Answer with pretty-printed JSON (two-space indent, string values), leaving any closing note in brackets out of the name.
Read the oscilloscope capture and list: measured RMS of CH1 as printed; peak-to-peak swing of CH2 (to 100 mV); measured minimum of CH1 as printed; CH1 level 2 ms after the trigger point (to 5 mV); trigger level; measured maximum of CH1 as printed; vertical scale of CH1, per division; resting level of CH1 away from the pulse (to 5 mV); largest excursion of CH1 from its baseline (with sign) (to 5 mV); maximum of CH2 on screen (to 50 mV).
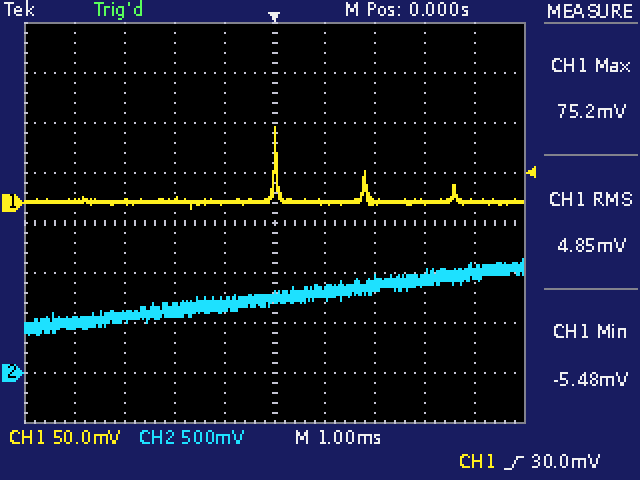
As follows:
{
  "measured RMS of CH1 as printed": "4.85 mV",
  "peak-to-peak swing of CH2": "800 mV",
  "measured minimum of CH1 as printed": "-5.48 mV",
  "CH1 level 2 ms after the trigger point": "0 mV",
  "trigger level": "30.0 mV",
  "measured maximum of CH1 as printed": "75.2 mV",
  "vertical scale of CH1, per division": "50 mV",
  "resting level of CH1 away from the pulse": "0 mV",
  "largest excursion of CH1 from its baseline (with sign)": "+75 mV",
  "maximum of CH2 on screen": "1.15 V"
}
